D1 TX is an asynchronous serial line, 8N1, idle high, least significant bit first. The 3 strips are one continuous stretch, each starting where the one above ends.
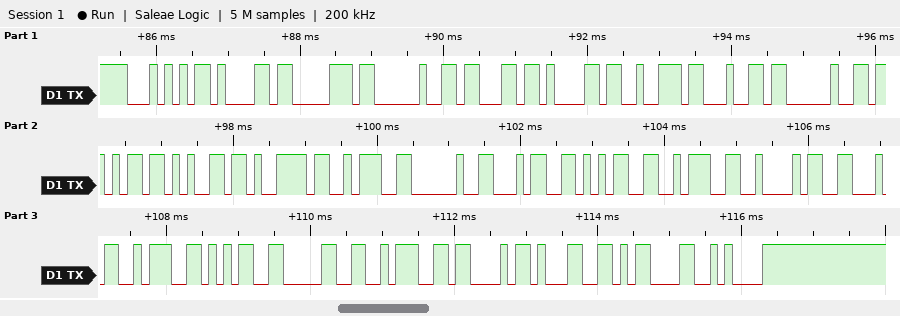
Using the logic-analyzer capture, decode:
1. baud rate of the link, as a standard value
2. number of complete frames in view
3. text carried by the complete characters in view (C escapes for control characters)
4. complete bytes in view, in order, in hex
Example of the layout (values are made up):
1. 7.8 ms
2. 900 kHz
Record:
1. 9600 baud
2. 27
3. "Tap card key: 45:BF:50:C1\r\n"
4. 54 61 70 20 63 61 72 64 20 6B 65 79 3A 20 34 35 3A 42 46 3A 35 30 3A 43 31 0D 0A
